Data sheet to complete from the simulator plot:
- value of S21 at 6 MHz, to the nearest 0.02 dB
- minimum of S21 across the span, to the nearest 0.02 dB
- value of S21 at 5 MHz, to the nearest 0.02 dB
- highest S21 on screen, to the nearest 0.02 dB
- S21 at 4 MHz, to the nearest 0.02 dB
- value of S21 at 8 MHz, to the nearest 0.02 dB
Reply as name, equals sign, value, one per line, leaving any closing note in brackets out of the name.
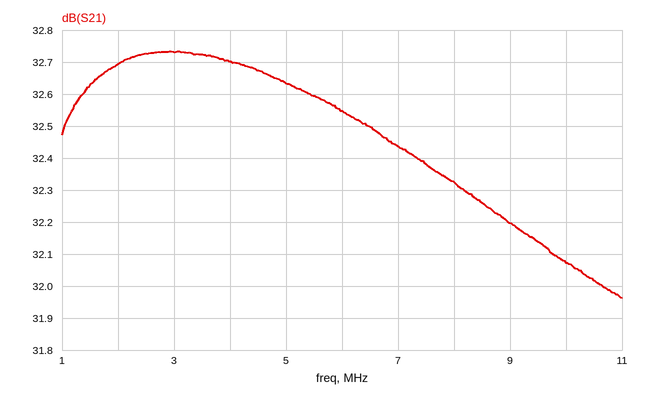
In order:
value of S21 at 6 MHz, to the nearest 0.02 dB = 32.54 dB
minimum of S21 across the span, to the nearest 0.02 dB = 31.96 dB
value of S21 at 5 MHz, to the nearest 0.02 dB = 32.64 dB
highest S21 on screen, to the nearest 0.02 dB = 32.74 dB
S21 at 4 MHz, to the nearest 0.02 dB = 32.70 dB
value of S21 at 8 MHz, to the nearest 0.02 dB = 32.32 dB
